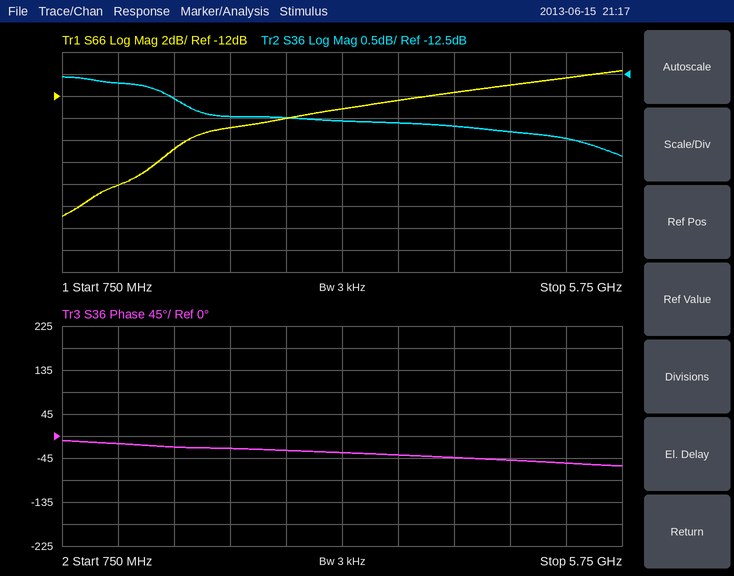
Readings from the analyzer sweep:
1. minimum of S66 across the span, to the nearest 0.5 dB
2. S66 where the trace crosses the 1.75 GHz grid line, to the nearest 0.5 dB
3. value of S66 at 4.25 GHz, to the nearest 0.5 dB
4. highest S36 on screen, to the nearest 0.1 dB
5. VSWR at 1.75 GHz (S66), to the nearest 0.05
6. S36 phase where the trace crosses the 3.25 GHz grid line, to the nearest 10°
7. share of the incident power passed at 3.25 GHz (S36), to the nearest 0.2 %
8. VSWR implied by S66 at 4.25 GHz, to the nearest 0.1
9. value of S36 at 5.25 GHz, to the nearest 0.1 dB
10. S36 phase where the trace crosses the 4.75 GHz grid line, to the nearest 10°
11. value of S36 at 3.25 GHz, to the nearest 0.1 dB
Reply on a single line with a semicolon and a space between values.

-23.0 dB; -17.0 dB; -11.5 dB; -12.6 dB; 1.35; -30°; 4.4 %; 1.7; -14.0 dB; -50°; -13.6 dB
